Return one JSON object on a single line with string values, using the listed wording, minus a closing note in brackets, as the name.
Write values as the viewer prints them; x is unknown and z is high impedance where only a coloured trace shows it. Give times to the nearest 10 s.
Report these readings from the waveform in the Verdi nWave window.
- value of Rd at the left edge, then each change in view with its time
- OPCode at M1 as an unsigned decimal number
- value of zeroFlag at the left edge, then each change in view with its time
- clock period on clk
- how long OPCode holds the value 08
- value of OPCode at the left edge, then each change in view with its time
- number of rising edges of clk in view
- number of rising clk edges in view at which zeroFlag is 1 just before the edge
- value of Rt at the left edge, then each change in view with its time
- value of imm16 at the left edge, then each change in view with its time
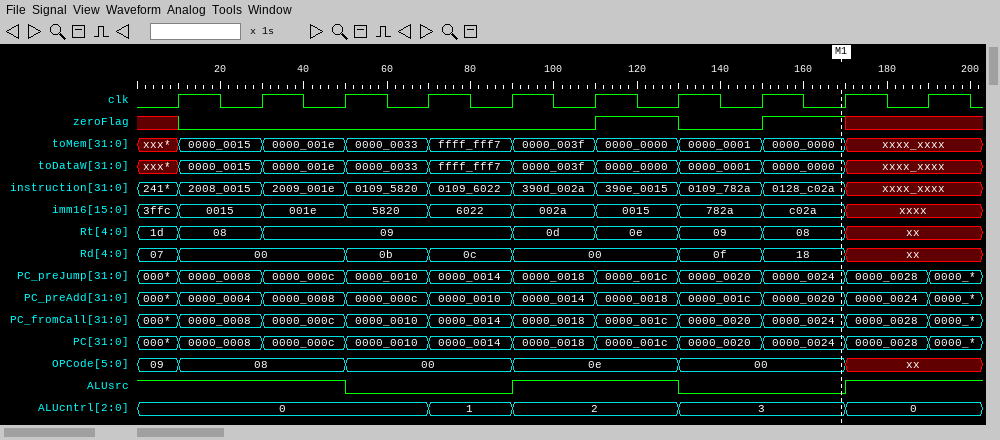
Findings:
{"value of Rd at the left edge, then each change in view with its time": "07, 00 at 10 s, 0b at 50 s, 0c at 70 s, 00 at 90 s, 0f at 130 s, 18 at 150 s, xx at 170 s", "OPCode at M1 as an unsigned decimal number": "0", "value of zeroFlag at the left edge, then each change in view with its time": "x, 0 at 10 s, 1 at 110 s, 0 at 130 s, 1 at 150 s, x at 170 s", "clock period on clk": "20 s", "how long OPCode holds the value 08": "40 s", "value of OPCode at the left edge, then each change in view with its time": "09, 08 at 10 s, 00 at 50 s, 0e at 90 s, 00 at 130 s, xx at 170 s", "number of rising edges of clk in view": "10", "number of rising clk edges in view at which zeroFlag is 1 just before the edge": "2", "value of Rt at the left edge, then each change in view with its time": "1d, 08 at 10 s, 09 at 30 s, 0d at 90 s, 0e at 110 s, 09 at 130 s, 08 at 150 s, xx at 170 s", "value of imm16 at the left edge, then each change in view with its time": "3ffc, 0015 at 10 s, 001e at 30 s, 5820 at 50 s, 6022 at 70 s, 002a at 90 s, 0015 at 110 s, 782a at 130 s, c02a at 150 s, xxxx at 170 s"}
